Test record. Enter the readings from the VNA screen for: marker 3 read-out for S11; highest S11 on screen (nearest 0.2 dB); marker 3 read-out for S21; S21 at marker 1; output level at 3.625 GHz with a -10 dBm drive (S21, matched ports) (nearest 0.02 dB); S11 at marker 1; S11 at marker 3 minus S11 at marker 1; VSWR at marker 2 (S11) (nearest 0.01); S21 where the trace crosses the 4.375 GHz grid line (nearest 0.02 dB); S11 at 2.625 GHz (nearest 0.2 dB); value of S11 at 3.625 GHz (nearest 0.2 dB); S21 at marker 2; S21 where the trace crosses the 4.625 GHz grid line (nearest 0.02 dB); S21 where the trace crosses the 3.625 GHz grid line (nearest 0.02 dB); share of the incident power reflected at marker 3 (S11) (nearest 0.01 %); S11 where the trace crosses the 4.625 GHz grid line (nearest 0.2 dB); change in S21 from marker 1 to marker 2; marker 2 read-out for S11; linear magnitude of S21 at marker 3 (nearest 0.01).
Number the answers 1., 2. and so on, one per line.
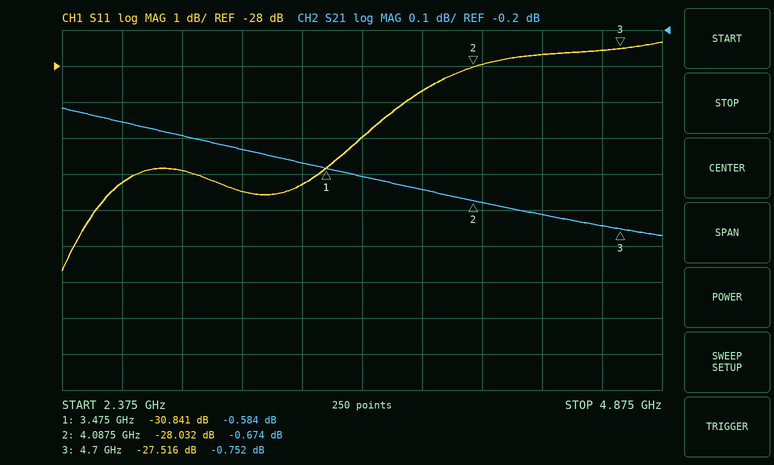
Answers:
1. -27.516 dB
2. -27.4 dB
3. -0.752 dB
4. -0.584 dB
5. -10.60 dBm
6. -30.841 dB
7. 3.325 dB
8. 1.08
9. -0.72 dB
10. -31.2 dB
11. -30.0 dB
12. -0.674 dB
13. -0.74 dB
14. -0.60 dB
15. 0.18 %
16. -27.6 dB
17. -0.090 dB
18. -28.032 dB
19. 0.92
